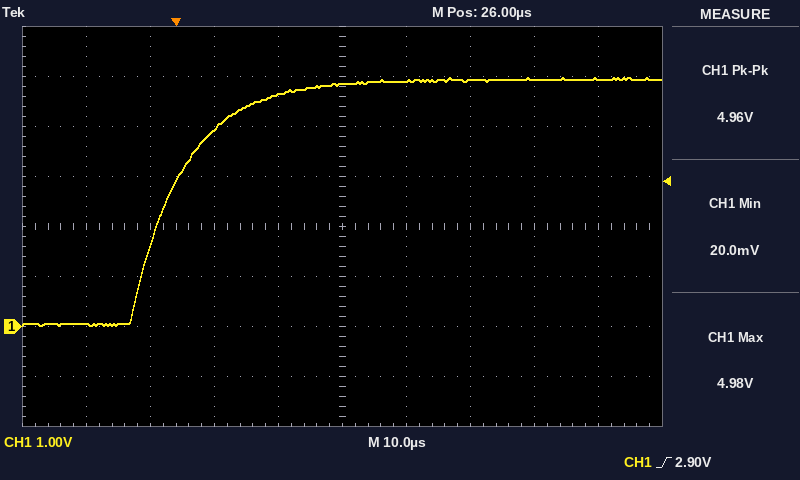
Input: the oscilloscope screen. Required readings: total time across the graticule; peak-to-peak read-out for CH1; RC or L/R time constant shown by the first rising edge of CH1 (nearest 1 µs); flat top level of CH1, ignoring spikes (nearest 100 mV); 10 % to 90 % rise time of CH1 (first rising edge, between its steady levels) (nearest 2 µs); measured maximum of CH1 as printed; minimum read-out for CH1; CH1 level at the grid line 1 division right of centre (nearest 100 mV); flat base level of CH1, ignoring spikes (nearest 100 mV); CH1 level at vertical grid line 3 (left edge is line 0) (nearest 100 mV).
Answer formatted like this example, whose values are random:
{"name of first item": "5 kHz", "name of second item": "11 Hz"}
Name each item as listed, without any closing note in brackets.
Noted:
{"total time across the graticule": "100 µs", "peak-to-peak read-out for CH1": "4.96 V", "RC or L/R time constant shown by the first rising edge of CH1": "8 µs", "flat top level of CH1, ignoring spikes": "4.9 V", "10 % to 90 % rise time of CH1 (first rising edge, between its steady levels)": "18 µs", "measured maximum of CH1 as printed": "4.98 V", "minimum read-out for CH1": "20.0 mV", "CH1 level at the grid line 1 division right of centre": "4.9 V", "flat base level of CH1, ignoring spikes": "100 mV", "CH1 level at vertical grid line 3 (left edge is line 0)": "3.9 V"}
